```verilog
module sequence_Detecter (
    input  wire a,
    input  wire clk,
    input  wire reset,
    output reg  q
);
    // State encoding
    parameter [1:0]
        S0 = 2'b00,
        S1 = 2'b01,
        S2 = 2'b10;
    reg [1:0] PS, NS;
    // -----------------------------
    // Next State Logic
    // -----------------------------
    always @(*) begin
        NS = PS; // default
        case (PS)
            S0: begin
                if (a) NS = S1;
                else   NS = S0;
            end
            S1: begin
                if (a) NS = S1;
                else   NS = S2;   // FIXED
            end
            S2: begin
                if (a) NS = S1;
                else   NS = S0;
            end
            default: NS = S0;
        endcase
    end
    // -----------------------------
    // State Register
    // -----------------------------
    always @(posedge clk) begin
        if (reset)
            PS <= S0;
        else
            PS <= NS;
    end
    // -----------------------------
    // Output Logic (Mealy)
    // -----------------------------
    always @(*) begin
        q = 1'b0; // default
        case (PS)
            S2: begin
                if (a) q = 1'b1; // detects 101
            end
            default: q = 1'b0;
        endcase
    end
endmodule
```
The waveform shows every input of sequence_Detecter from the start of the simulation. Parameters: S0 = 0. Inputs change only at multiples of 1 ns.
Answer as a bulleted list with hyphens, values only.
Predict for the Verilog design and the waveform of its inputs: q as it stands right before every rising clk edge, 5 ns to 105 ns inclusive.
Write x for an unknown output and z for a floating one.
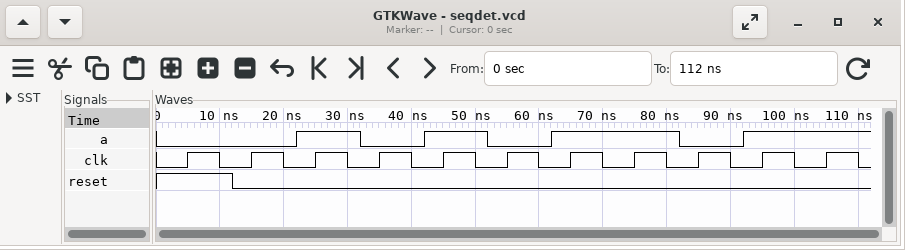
- 0 0 0 0 1 0 1 0 0 1 0
